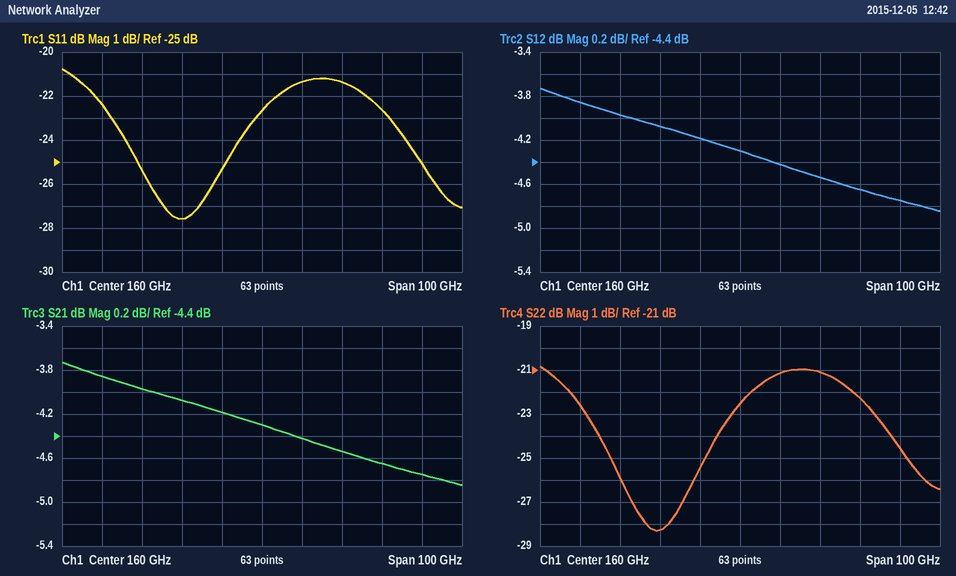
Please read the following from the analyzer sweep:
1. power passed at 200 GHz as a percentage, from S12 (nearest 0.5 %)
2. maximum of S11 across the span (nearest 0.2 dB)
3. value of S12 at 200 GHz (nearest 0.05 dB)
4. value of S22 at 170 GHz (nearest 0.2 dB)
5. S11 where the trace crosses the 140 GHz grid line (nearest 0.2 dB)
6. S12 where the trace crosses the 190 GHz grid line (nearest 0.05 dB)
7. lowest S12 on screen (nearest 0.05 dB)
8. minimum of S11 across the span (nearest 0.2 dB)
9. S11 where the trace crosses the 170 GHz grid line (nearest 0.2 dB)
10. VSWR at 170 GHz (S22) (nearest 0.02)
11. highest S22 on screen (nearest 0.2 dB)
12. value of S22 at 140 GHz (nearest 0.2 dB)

33.5 %
-20.8 dB
-4.75 dB
-21.2 dB
-27.6 dB
-4.65 dB
-4.85 dB
-27.6 dB
-21.4 dB
1.20
-20.8 dB
-28.2 dB
